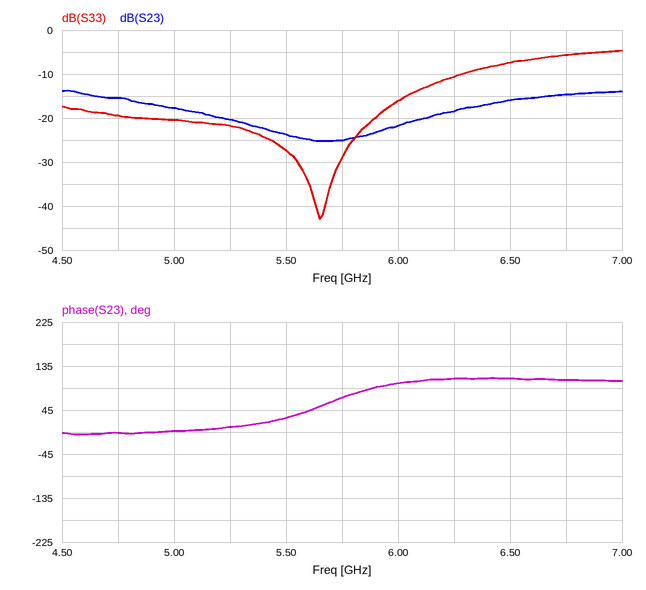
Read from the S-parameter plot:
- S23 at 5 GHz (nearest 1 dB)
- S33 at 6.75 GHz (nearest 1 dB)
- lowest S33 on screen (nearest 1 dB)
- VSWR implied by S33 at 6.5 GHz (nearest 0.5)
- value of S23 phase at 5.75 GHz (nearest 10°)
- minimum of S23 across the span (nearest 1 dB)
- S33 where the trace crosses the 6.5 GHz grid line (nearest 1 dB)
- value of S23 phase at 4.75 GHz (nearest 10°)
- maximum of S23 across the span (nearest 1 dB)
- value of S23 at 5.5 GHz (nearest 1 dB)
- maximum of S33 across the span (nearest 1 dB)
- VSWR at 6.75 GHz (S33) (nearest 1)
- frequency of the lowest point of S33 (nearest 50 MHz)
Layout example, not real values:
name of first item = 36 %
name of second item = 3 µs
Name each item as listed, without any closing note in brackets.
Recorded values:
S23 at 5 GHz = -18 dB
S33 at 6.75 GHz = -6 dB
lowest S33 on screen = -43 dB
VSWR implied by S33 at 6.5 GHz = 2.5
value of S23 phase at 5.75 GHz = 70°
minimum of S23 across the span = -25 dB
S33 where the trace crosses the 6.5 GHz grid line = -7 dB
value of S23 phase at 4.75 GHz = 0°
maximum of S23 across the span = -14 dB
value of S23 at 5.5 GHz = -24 dB
maximum of S33 across the span = -5 dB
VSWR at 6.75 GHz (S33) = 3
frequency of the lowest point of S33 = 5.65 GHz
